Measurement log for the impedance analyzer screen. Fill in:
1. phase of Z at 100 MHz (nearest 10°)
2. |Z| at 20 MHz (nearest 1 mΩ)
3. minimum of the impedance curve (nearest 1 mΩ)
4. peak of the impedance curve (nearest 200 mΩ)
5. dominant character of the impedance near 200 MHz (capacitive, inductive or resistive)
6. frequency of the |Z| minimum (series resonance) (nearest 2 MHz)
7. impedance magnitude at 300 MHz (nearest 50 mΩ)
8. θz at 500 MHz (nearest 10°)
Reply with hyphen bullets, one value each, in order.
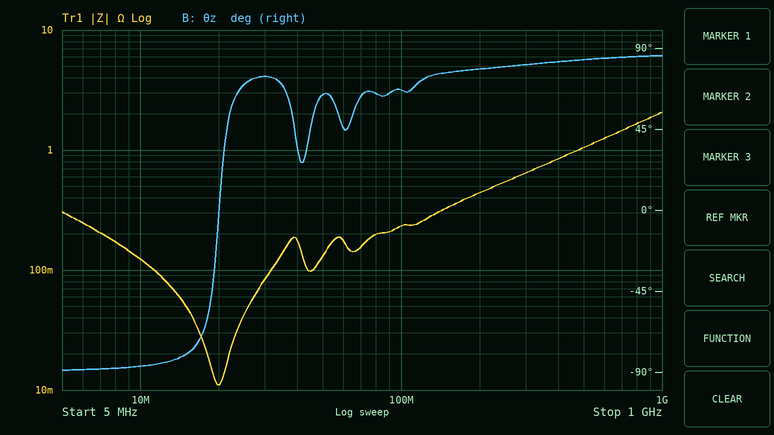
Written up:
- 70°
- 11 mΩ
- 11 mΩ
- 2.0 Ω
- inductive
- 20 MHz
- 650 mΩ
- 80°
